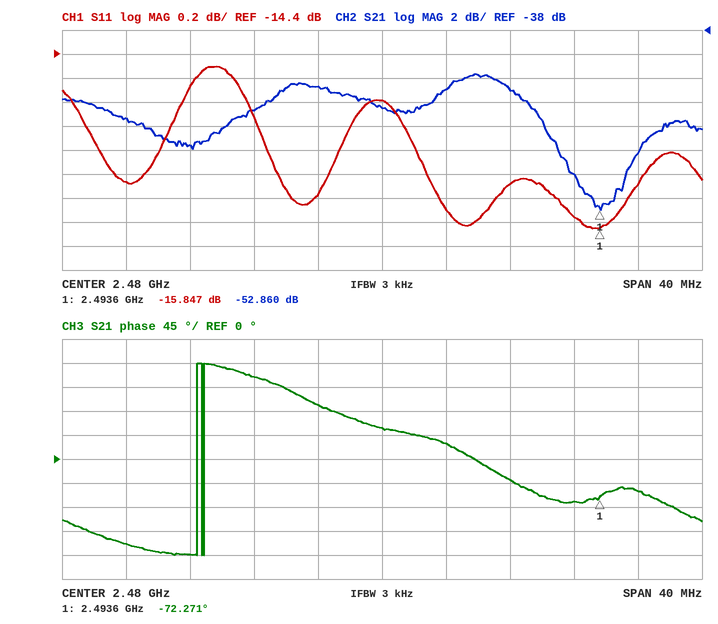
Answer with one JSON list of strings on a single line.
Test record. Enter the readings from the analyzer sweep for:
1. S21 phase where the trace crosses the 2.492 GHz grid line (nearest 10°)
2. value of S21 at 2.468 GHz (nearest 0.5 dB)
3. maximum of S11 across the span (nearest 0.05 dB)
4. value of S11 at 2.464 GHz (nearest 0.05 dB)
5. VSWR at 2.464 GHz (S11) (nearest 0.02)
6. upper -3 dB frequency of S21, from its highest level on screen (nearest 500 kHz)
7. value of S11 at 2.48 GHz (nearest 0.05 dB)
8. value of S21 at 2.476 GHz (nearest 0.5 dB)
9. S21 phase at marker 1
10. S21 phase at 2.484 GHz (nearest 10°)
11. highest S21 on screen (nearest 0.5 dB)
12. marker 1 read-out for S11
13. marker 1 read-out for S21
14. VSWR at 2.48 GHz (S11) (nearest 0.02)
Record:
["-80°", "-47.5 dB", "-14.50 dB", "-15.45 dB", "1.40", "2.4895 GHz", "-14.80 dB", "-42.5 dB", "-72.271°", "30°", "-41.5 dB", "-15.847 dB", "-52.860 dB", "1.44"]
